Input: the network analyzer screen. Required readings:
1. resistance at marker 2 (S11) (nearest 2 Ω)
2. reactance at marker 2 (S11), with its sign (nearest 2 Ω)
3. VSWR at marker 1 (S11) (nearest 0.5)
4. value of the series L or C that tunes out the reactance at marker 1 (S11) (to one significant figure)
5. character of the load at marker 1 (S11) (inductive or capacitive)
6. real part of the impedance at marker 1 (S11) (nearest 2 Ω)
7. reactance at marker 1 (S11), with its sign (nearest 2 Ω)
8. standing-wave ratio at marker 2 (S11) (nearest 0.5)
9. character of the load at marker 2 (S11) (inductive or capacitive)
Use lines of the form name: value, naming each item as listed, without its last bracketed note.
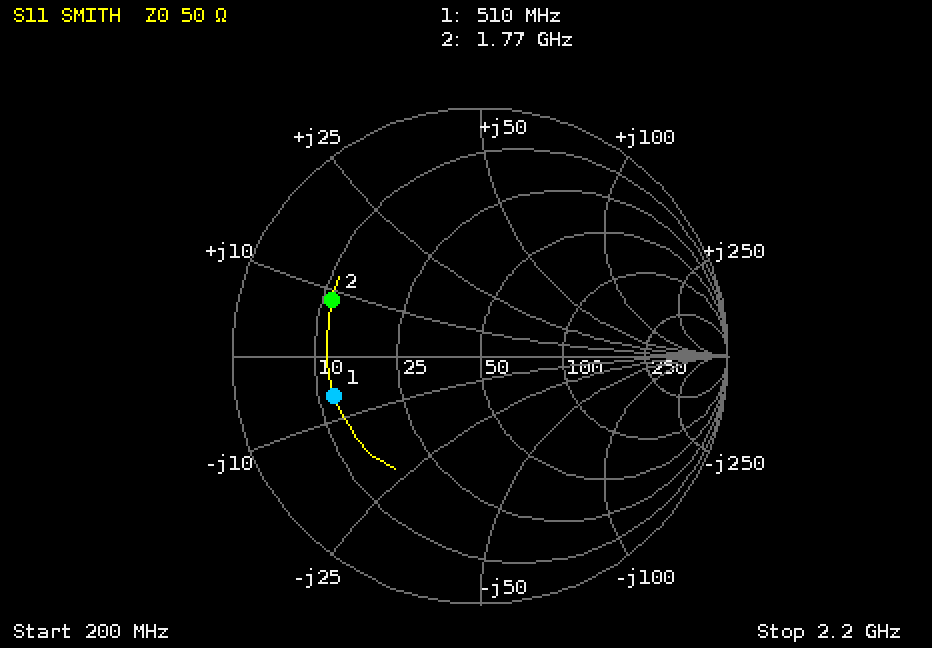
resistance at marker 2 (S11): 12 Ω
reactance at marker 2 (S11), with its sign: +8 Ω
VSWR at marker 1 (S11): 4.0
value of the series L or C that tunes out the reactance at marker 1 (S11): 2 nH
character of the load at marker 1 (S11): capacitive
real part of the impedance at marker 1 (S11): 12 Ω
reactance at marker 1 (S11), with its sign: -6 Ω
standing-wave ratio at marker 2 (S11): 4.5
character of the load at marker 2 (S11): inductive
